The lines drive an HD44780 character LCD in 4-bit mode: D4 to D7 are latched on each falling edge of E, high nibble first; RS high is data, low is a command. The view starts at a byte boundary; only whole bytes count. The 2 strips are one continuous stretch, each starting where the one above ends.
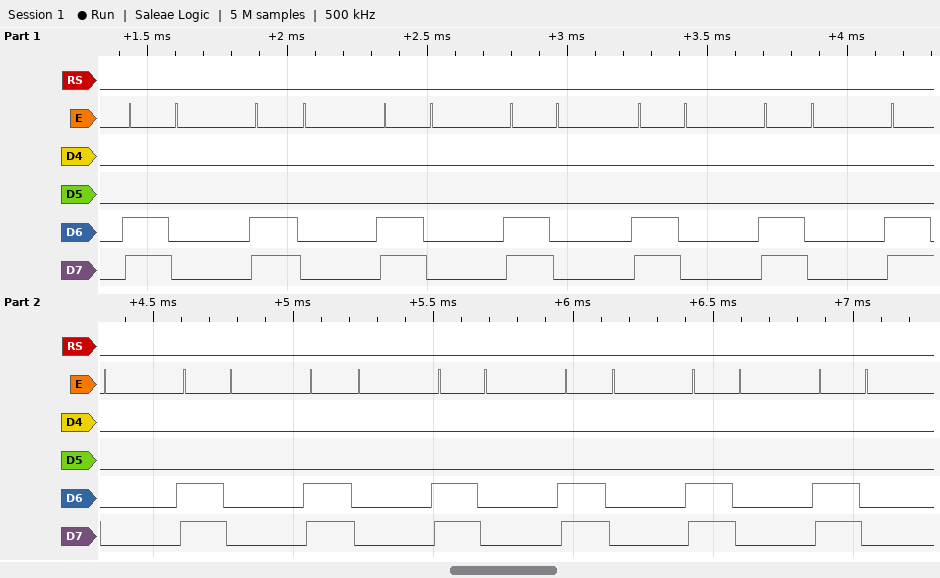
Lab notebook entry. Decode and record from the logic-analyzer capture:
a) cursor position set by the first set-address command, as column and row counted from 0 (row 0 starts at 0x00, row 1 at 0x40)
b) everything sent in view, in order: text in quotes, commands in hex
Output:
column 0, row 1
0xC0 0xC0 0xC0 0xC0 0xC0 0xC0 0xC0 0xC0 0xC0 0xC0 0xC0 0xC0 0xC0
